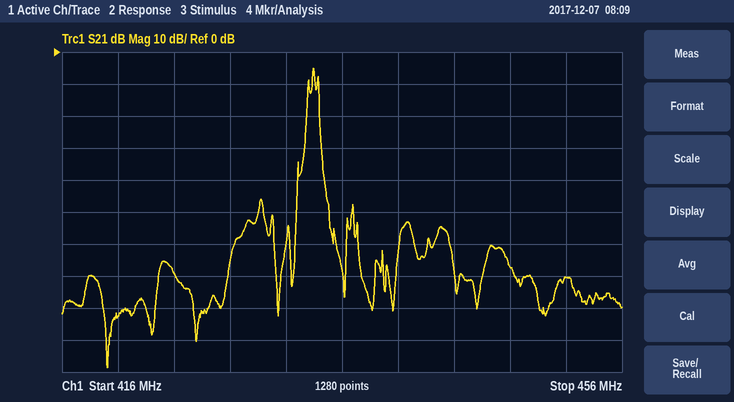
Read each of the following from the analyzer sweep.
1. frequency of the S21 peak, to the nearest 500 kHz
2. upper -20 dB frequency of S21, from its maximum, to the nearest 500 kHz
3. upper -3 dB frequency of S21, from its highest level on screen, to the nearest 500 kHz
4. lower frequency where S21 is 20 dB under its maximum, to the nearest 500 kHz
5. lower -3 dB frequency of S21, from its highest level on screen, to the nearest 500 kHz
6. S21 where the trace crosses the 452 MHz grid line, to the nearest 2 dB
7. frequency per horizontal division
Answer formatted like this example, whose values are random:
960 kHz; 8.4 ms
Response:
434.0 MHz; 434.5 MHz; 434.0 MHz; 433.5 MHz; 434.0 MHz; -70 dB; 4 MHz
